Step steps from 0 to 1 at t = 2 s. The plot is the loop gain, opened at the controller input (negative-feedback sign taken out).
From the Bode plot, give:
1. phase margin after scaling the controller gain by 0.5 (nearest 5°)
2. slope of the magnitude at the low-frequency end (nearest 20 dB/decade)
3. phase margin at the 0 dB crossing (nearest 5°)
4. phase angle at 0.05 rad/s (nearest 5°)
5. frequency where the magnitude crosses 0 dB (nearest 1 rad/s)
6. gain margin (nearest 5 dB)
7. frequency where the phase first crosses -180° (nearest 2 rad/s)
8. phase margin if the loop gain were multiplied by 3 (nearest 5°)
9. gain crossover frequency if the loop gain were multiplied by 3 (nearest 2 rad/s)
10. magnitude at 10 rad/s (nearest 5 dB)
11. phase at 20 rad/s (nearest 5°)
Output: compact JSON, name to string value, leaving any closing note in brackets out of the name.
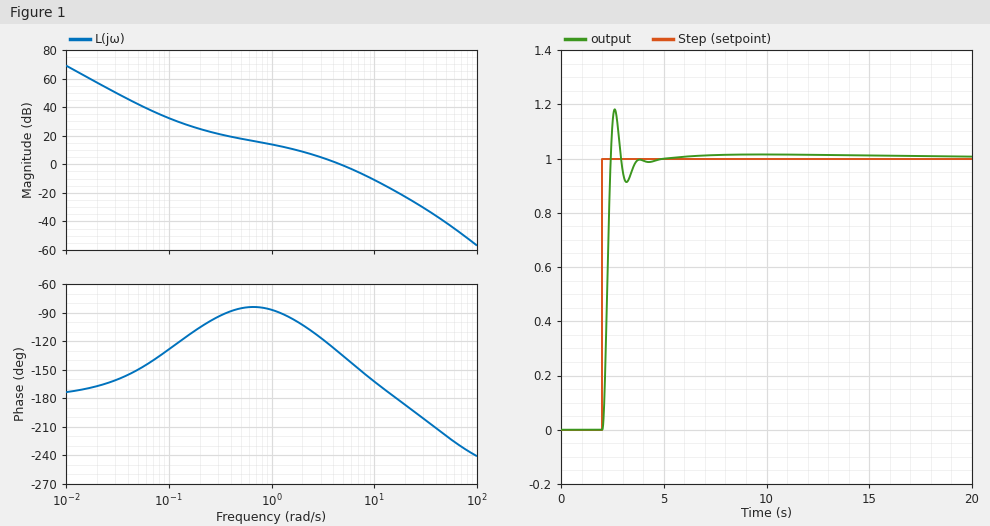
{"phase margin after scaling the controller gain by 0.5": "65°", "slope of the magnitude at the low-frequency end": "-40 dB/decade", "phase margin at the 0 dB crossing": "45°", "phase angle at 0.05 rad/s": "-150°", "frequency where the magnitude crosses 0 dB": "5 rad/s", "gain margin": "20 dB", "frequency where the phase first crosses -180°": "16 rad/s", "phase margin if the loop gain were multiplied by 3": "20°", "gain crossover frequency if the loop gain were multiplied by 3": "10 rad/s", "magnitude at 10 rad/s": "-10 dB", "phase at 20 rad/s": "-185°"}
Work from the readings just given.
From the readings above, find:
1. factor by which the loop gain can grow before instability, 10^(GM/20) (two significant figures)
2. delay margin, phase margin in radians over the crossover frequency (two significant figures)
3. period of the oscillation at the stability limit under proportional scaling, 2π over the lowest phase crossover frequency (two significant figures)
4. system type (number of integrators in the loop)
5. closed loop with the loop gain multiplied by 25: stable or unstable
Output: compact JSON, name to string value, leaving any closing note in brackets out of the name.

{"factor by which the loop gain can grow before instability, 10^(GM/20)": "10", "delay margin, phase margin in radians over the crossover frequency": "0.16 s", "period of the oscillation at the stability limit under proportional scaling, 2π over the lowest phase crossover frequency": "0.39 s", "system type": "2", "closed loop with the loop gain multiplied by 25: stable or unstable": "unstable"}
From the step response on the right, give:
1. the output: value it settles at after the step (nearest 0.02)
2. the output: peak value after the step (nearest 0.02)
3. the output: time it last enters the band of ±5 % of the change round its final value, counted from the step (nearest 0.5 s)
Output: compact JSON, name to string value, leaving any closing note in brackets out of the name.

{"the output: value it settles at after the step": "1.00", "the output: peak value after the step": "1.18", "the output: time it last enters the band of ±5 % of the change round its final value, counted from the step": "1.5 s"}
